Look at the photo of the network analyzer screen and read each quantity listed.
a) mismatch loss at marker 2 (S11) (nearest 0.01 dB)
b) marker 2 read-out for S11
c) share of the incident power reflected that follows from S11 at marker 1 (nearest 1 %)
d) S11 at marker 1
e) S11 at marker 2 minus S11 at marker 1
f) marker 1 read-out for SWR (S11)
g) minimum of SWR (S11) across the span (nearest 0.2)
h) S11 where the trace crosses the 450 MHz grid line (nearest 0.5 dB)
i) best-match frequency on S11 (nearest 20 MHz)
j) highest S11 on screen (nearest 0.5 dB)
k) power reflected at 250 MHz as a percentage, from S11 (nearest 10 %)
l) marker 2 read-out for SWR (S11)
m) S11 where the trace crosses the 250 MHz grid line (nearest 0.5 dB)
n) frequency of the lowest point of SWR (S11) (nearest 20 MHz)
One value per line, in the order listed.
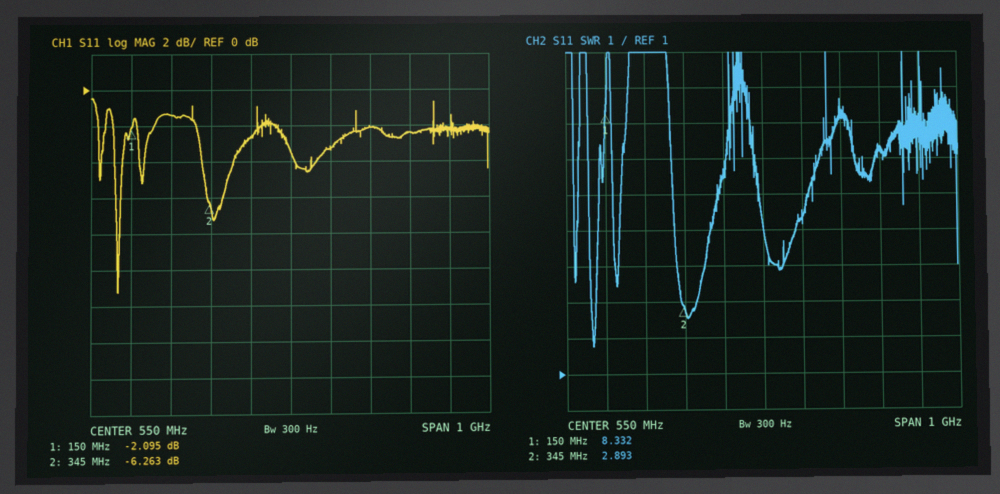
1.17 dB
-6.263 dB
62 %
-2.095 dB
-4.168 dB
8.332
1.8
-2.5 dB
120 MHz
-0.5 dB
70 %
2.893
-1.5 dB
120 MHz
